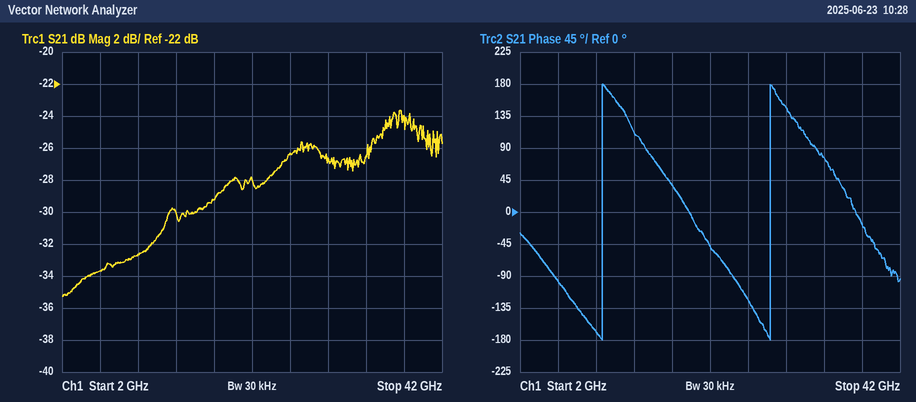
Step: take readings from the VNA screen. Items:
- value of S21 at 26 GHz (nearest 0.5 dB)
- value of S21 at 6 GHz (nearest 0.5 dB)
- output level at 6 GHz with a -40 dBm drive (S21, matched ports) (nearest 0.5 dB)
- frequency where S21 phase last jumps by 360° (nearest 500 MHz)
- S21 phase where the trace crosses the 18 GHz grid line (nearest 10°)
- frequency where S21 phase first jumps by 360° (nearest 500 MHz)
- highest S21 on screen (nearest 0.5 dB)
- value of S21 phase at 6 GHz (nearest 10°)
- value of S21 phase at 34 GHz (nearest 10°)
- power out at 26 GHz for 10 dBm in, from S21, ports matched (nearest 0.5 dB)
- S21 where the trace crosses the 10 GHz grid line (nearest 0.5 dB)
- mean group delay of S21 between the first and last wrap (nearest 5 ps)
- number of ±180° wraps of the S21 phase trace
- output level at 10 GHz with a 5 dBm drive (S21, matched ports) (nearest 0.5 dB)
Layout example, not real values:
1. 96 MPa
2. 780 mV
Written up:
1. -26.5 dB
2. -33.5 dB
3. -73.5 dBm
4. 28.5 GHz
5. 40°
6. 10.5 GHz
7. -23.5 dB
8. -100°
9. 80°
10. -16.5 dBm
11. -32.5 dB
12. 55 ps
13. 2
14. -27.5 dBm
